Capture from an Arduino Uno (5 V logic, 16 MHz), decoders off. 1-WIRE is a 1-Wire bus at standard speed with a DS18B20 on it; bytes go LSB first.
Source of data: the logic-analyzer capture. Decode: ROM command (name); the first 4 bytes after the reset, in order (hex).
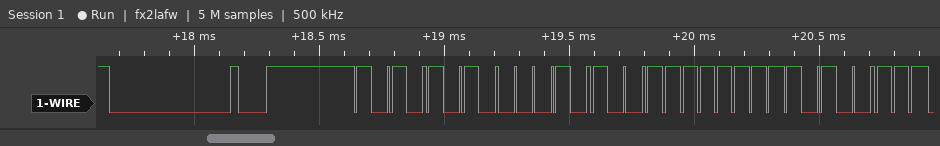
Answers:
Match ROM
55 28 FF E5
